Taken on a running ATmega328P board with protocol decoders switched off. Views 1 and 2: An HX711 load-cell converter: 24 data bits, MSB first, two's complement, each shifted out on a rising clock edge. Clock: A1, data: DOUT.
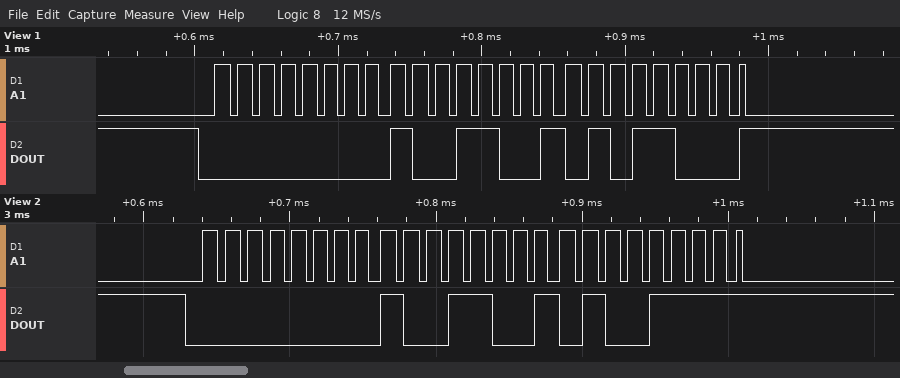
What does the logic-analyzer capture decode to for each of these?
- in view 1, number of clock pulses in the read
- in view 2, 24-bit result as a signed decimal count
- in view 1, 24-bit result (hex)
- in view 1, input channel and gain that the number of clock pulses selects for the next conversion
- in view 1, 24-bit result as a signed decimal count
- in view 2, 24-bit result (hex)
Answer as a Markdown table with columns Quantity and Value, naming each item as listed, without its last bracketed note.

| Quantity | Value |
|---|---|
| in view 1, number of clock pulses in the read | 25 |
| in view 2, 24-bit result as a signed decimal count | 39247 |
| in view 1, 24-bit result | 0x009958 |
| in view 1, input channel and gain that the number of clock pulses selects for the next conversion | channel A, gain 128 |
| in view 1, 24-bit result as a signed decimal count | 39256 |
| in view 2, 24-bit result | 0x00994F |
